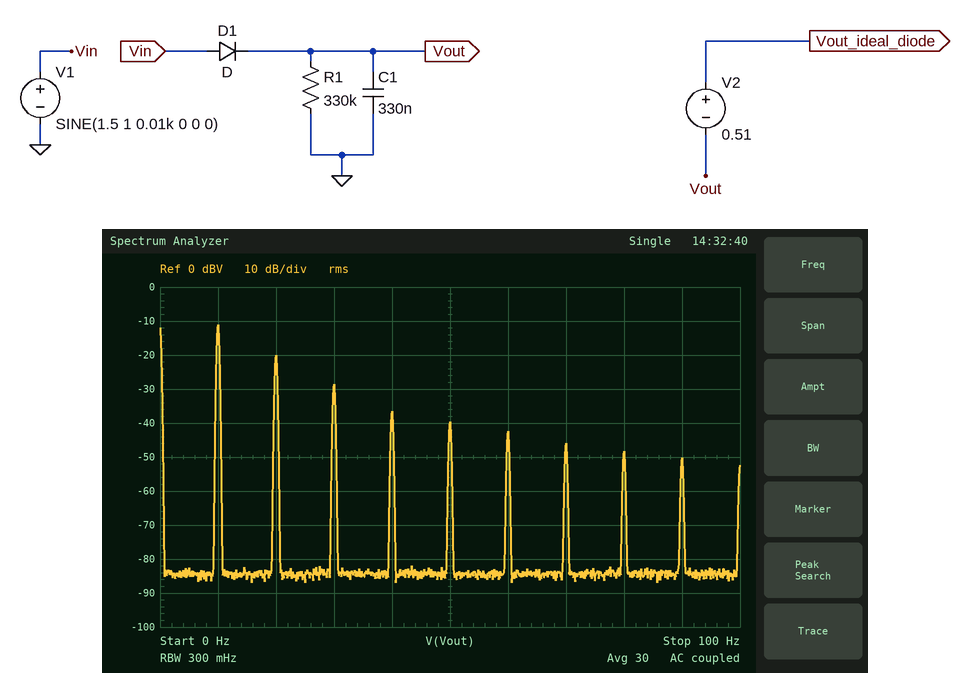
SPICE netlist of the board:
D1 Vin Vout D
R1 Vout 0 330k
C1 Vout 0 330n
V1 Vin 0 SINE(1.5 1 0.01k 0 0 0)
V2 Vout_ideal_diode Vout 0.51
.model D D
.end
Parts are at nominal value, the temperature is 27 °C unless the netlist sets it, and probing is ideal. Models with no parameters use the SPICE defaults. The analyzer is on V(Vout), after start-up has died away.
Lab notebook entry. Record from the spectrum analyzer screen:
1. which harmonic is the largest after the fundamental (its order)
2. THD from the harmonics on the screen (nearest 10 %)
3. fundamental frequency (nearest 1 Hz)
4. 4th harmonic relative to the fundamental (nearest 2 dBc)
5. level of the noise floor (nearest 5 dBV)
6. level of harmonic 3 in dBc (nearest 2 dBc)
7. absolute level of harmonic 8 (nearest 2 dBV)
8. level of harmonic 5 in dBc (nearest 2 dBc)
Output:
2
40 %
10 Hz
-26 dBc
-85 dBV
-18 dBc
-48 dBV
-28 dBc
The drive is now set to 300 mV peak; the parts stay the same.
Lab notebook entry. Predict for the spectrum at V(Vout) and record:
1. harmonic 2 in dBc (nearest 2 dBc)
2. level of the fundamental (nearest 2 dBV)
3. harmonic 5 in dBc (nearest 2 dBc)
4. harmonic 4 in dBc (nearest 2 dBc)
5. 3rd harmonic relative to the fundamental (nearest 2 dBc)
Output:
-14 dBc
-16 dBV
-36 dBc
-32 dBc
-26 dBc
